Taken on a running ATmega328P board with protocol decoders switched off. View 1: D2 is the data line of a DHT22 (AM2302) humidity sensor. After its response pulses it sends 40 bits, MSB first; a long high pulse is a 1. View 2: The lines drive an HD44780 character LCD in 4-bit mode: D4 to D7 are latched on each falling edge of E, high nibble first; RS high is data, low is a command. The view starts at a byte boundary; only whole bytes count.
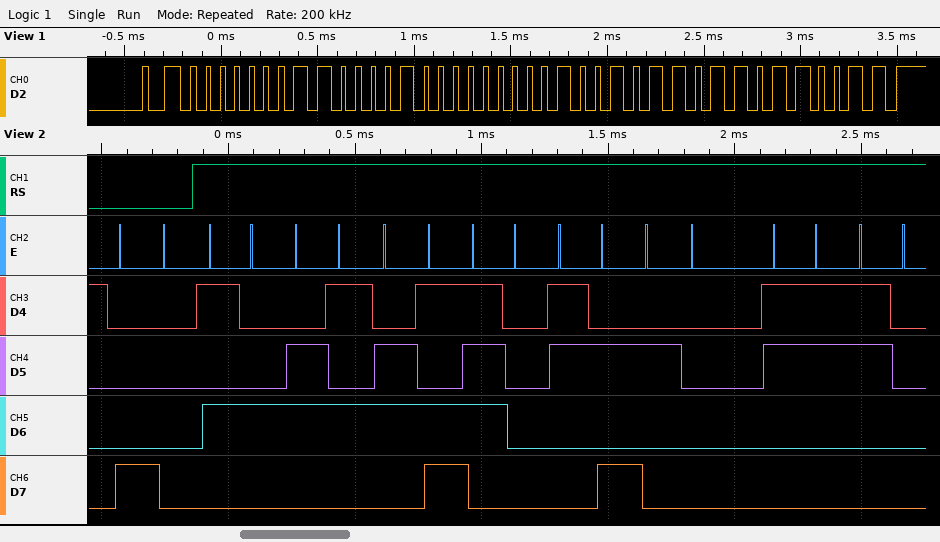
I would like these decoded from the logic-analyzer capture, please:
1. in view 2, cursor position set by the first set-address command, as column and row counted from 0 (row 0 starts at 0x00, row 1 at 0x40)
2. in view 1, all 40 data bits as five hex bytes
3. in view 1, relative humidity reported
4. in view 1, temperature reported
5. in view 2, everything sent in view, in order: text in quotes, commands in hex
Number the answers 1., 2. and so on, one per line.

1. column 0, row 0
2. 01 84 01 2D B3
3. 38.8 %
4. 30.1 °C
5. 0x80 "Temp: 30"
